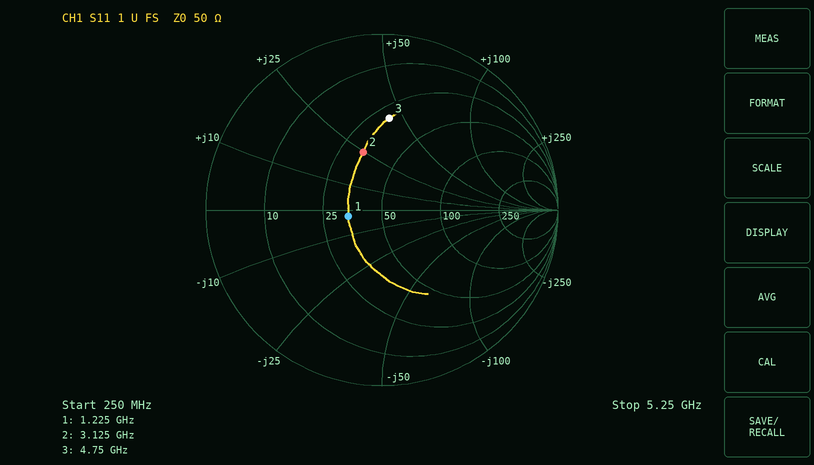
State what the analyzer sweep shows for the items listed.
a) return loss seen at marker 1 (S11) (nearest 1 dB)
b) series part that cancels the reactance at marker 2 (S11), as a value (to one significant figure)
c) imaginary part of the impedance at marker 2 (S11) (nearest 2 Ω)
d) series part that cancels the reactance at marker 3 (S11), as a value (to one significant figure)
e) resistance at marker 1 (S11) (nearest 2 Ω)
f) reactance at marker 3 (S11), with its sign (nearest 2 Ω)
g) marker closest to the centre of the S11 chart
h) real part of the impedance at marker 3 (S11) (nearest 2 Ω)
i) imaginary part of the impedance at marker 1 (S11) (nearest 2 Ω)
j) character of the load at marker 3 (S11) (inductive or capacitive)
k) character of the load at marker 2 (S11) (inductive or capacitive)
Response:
14 dB
2 pF
+24 Ω
800 fF
34 Ω
+44 Ω
marker 1
30 Ω
-2 Ω
inductive
inductive
